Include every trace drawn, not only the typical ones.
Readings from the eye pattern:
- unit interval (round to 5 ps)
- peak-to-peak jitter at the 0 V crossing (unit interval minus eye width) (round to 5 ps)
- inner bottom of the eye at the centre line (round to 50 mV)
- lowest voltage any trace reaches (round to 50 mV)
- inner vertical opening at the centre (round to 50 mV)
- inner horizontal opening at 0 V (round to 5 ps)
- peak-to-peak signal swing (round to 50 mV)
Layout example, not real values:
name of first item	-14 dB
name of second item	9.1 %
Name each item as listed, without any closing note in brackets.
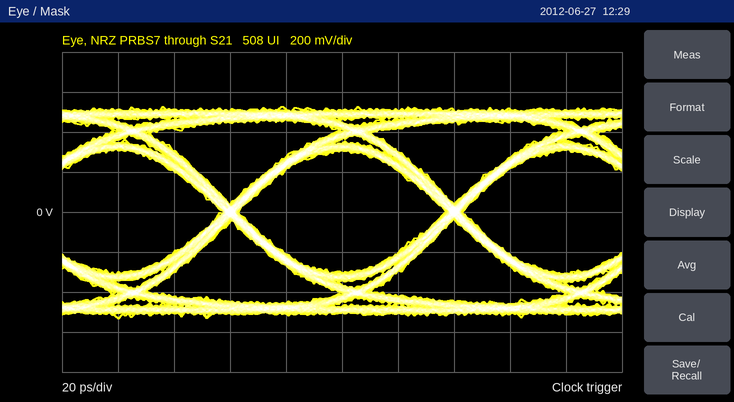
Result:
unit interval	80 ps
peak-to-peak jitter at the 0 V crossing (unit interval minus eye width)	5 ps
inner bottom of the eye at the centre line	-300 mV
lowest voltage any trace reaches	-550 mV
inner vertical opening at the centre	600 mV
inner horizontal opening at 0 V	75 ps
peak-to-peak signal swing	1.05 V
